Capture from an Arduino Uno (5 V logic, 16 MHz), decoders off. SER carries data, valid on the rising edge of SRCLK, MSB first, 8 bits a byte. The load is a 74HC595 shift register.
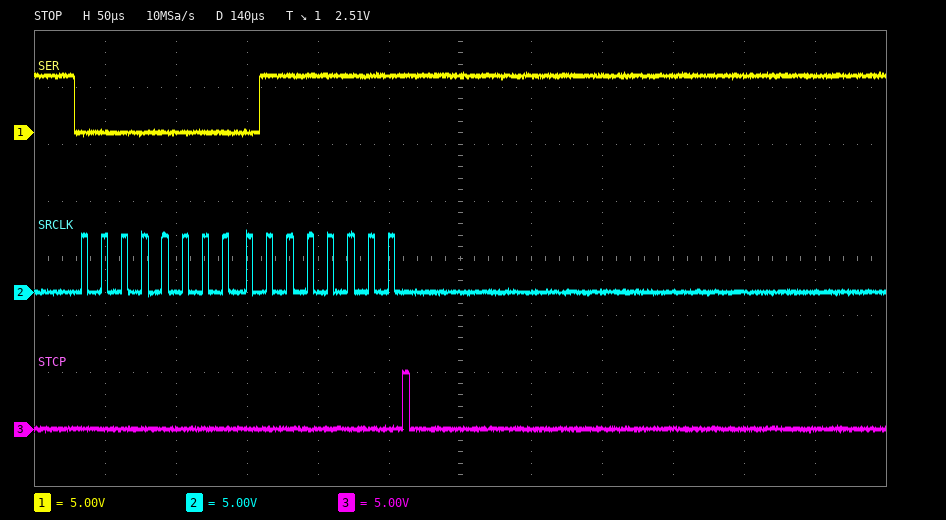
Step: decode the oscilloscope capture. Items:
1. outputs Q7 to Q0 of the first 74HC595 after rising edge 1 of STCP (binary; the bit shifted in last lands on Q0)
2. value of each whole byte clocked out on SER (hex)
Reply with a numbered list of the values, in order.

1. 01111111
2. 00 7F
